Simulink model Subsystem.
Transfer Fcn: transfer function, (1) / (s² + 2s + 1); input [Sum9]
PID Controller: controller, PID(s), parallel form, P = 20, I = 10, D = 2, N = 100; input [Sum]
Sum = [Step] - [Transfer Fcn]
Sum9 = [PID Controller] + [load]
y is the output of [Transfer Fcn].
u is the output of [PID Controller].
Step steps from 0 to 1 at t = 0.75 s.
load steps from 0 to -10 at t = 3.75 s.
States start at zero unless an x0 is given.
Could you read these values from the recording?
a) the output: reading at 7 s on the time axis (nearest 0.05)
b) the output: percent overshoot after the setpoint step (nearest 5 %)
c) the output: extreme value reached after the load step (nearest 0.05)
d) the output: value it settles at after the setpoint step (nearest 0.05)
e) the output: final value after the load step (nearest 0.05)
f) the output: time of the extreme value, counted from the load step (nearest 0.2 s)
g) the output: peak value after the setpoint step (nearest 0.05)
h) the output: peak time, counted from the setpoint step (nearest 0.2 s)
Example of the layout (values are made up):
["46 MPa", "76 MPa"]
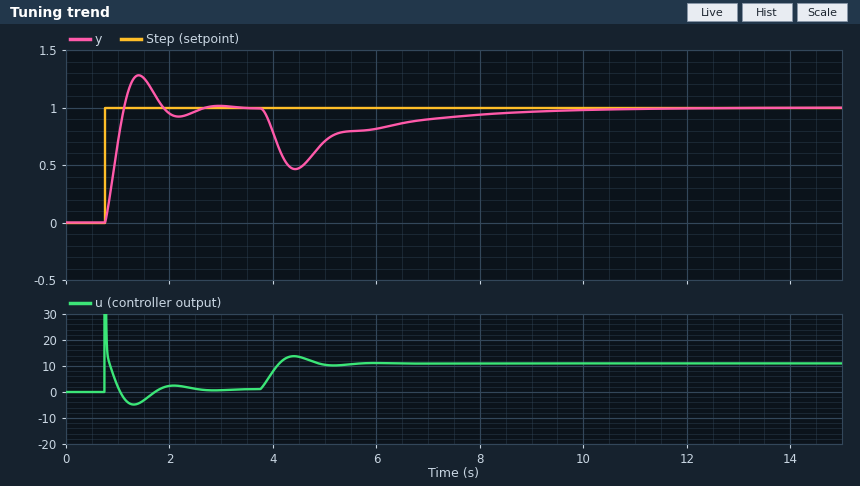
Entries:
["0.90", "30 %", "0.45", "1.00", "1.00", "0.6 s", "1.30", "0.6 s"]
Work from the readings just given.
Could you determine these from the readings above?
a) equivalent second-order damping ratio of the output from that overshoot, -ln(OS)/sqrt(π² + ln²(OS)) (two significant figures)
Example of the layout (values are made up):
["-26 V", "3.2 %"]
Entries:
["0.36"]
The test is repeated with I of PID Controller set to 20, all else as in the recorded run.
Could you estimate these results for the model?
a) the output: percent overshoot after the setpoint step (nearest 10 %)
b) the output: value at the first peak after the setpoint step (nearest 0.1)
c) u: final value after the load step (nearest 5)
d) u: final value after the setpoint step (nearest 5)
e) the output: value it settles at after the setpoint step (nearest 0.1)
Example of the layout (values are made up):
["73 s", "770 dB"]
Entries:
["40 %", "1.4", "10", "0", "1.0"]
